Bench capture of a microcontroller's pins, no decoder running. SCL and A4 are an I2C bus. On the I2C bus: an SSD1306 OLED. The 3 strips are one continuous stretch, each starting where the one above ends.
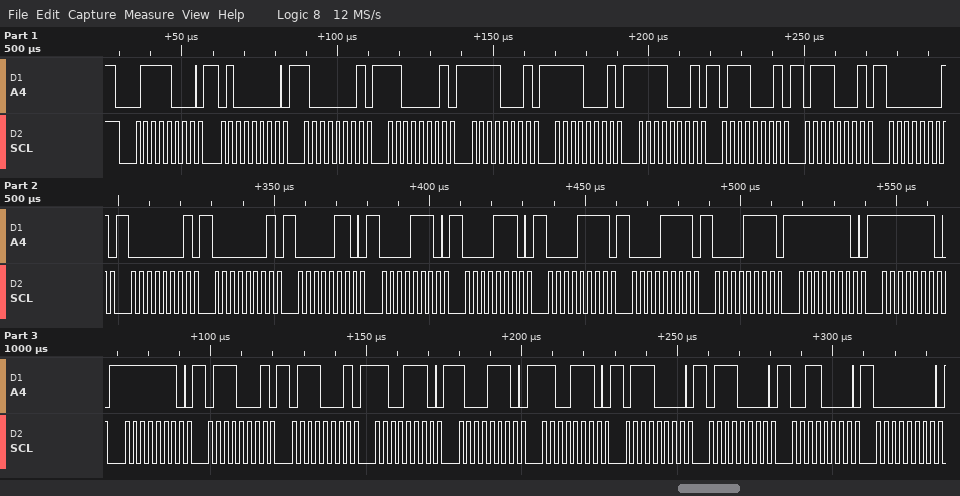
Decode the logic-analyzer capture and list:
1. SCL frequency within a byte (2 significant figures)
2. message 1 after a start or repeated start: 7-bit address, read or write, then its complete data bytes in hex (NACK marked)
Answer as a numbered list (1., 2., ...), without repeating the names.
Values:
1. 400 kHz
2. 0x3C write: 40 81 C1 F1 F1 F1 71 71 01 01 01 06 0E 0E 0F 0F 0F FE FE FE 71 71 CE 8E CE 70 70 30 00
